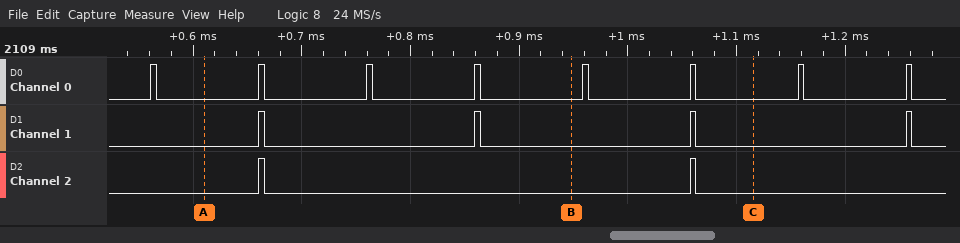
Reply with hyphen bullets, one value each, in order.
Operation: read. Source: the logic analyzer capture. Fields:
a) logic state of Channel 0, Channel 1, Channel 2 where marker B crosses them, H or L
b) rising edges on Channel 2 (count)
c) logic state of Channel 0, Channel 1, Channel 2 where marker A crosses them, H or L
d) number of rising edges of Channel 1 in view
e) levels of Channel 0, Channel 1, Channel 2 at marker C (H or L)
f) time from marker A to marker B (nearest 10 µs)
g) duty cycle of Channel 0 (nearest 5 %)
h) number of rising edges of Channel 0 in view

- Channel 0=L, Channel 1=L, Channel 2=L
- 2
- Channel 0=L, Channel 1=L, Channel 2=L
- 4
- Channel 0=L, Channel 1=L, Channel 2=L
- 340 µs
- 5 %
- 8
